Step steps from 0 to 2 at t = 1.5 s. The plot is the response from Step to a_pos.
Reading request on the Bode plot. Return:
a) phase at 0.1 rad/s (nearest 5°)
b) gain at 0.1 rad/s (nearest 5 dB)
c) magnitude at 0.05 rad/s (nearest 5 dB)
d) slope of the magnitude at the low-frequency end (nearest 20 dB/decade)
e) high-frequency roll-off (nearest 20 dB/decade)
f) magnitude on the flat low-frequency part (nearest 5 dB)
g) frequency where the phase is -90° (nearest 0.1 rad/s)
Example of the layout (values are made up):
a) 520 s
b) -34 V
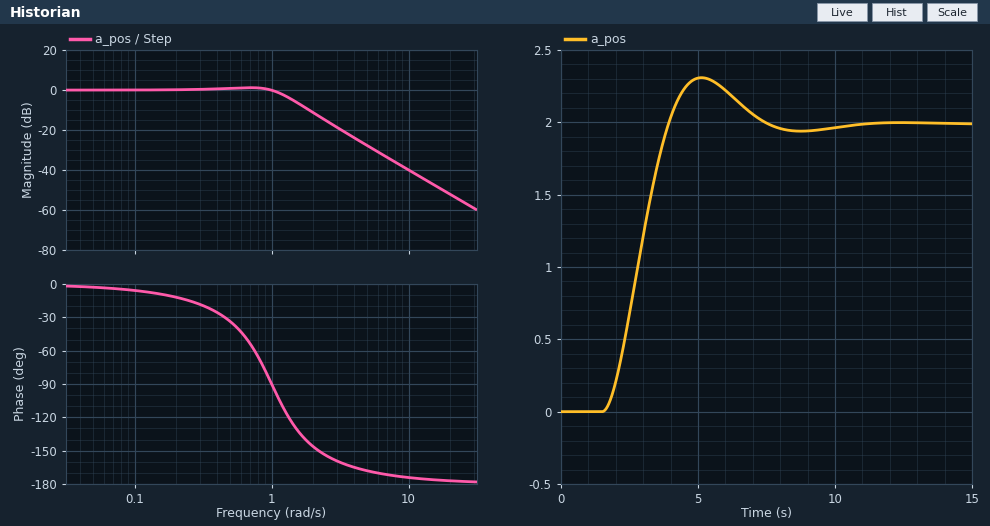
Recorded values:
a) -5°
b) 0 dB
c) 0 dB
d) 0 dB/decade
e) -40 dB/decade
f) 0 dB
g) 1.0 rad/s
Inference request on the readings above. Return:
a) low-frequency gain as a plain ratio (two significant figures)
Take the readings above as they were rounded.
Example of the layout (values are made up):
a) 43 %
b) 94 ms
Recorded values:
a) 1.0
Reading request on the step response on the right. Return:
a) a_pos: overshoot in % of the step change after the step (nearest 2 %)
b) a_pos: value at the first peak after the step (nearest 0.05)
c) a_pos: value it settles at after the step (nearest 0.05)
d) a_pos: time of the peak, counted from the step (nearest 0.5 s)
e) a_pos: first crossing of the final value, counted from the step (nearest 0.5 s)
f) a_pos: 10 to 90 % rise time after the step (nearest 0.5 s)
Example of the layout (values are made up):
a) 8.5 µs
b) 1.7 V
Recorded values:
a) 16 %
b) 2.30
c) 2.00
d) 3.5 s
e) 2.5 s
f) 1.5 s
